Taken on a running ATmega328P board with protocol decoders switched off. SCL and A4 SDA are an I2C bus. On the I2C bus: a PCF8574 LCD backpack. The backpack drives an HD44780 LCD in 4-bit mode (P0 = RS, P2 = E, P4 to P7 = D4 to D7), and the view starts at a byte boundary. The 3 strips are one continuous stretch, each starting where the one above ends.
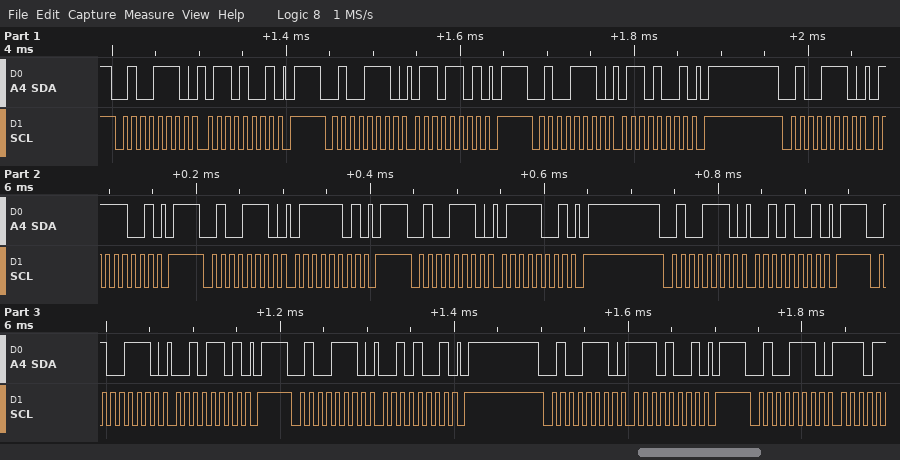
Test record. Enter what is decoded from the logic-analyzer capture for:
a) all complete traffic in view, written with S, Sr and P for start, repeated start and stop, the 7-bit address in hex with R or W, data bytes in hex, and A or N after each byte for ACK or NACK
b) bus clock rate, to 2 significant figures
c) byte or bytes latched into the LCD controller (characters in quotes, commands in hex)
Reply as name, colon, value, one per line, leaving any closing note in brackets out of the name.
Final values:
all complete traffic in view, written with S, Sr and P for start, repeated start and stop, the 7-bit address in hex with R or W, data bytes in hex, and A or N after each byte for ACK or NACK: S 27W A 69 A P S 27W A 6D A P S 27W A 69 A P S 27W A 79 A P S 27W A 7D A P S 27W A 79 A P S 27W A 29 A P S 27W A 2D A P S 27W A 29 A P S 27W A E9 A P S 27W A
bus clock rate, to 2 significant figures: 100 kHz
byte or bytes latched into the LCD controller: 'g'
